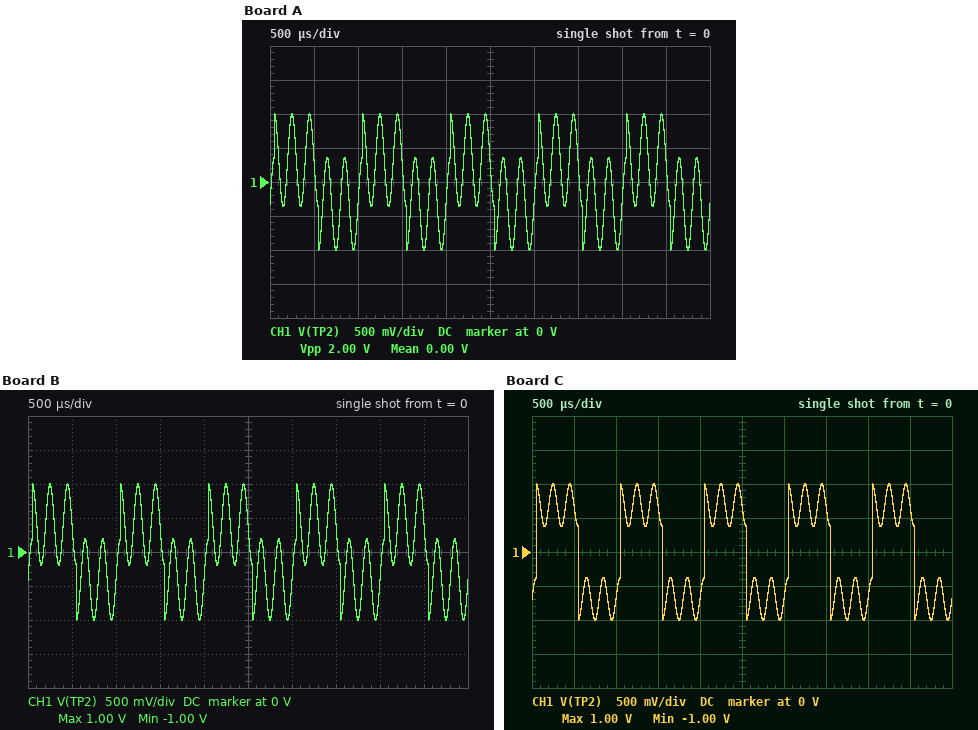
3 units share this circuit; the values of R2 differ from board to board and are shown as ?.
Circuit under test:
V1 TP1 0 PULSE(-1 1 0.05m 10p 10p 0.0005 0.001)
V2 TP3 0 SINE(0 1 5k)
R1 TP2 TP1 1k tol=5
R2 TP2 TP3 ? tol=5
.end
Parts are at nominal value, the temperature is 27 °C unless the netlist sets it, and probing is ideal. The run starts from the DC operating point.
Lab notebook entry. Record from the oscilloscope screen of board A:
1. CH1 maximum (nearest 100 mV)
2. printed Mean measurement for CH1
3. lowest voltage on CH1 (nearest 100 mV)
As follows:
1.0 V
0.00 V
-1.0 V
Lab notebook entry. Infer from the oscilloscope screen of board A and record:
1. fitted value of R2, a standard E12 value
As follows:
470 Ω
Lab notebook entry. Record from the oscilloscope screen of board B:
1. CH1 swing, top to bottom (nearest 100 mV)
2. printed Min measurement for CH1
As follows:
2.0 V
-1.00 V
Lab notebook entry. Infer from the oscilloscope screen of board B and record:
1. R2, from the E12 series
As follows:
680 Ω
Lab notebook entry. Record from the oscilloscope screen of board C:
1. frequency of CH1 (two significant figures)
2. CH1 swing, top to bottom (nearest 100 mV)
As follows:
1.0 kHz
2.0 V
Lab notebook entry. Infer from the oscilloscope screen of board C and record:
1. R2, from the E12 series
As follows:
2.2 kΩ
